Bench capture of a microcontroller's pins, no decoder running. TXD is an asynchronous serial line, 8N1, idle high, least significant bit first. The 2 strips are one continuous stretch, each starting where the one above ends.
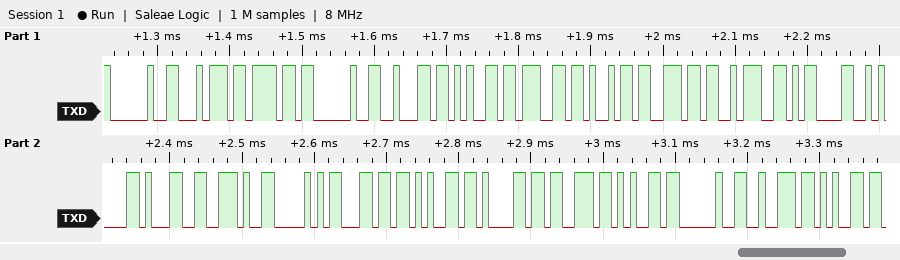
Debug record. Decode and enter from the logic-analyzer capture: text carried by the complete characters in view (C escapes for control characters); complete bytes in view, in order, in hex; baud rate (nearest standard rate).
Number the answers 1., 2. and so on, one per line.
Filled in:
1. " to begin:\r\n1.Please re"
2. 0x20 0x74 0x6F 0x20 0x62 0x65 0x67 0x69 0x6E 0x3A 0x0D 0x0A 0x31 0x2E 0x50 0x6C 0x65 0x61 0x73 0x65 0x20 0x72 0x65
3. 115200 baud
